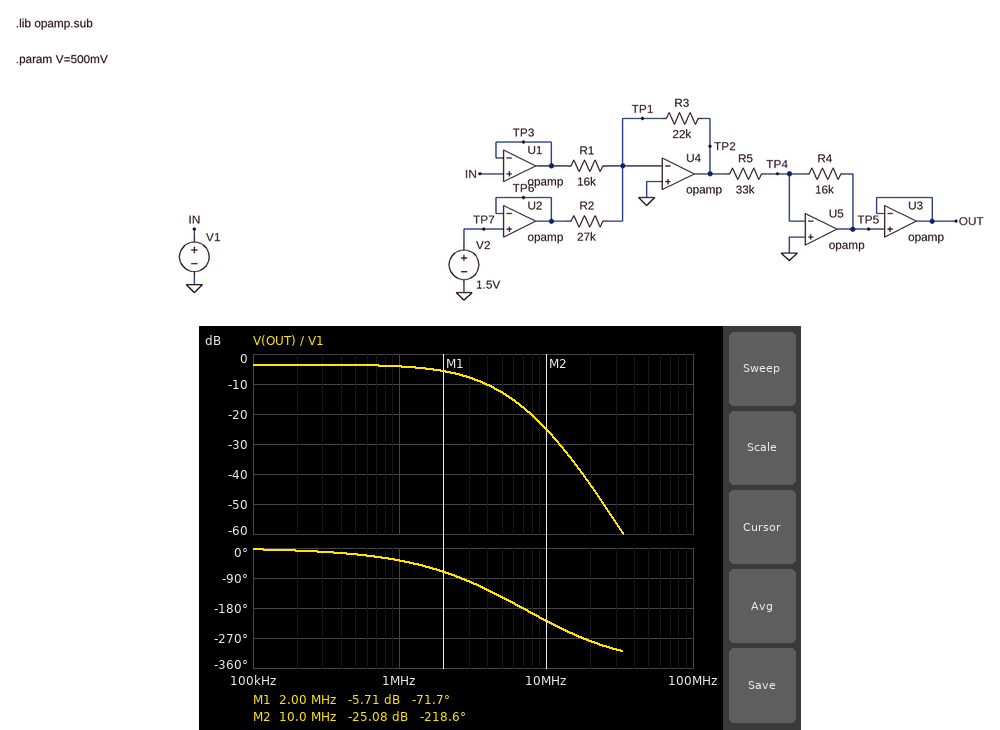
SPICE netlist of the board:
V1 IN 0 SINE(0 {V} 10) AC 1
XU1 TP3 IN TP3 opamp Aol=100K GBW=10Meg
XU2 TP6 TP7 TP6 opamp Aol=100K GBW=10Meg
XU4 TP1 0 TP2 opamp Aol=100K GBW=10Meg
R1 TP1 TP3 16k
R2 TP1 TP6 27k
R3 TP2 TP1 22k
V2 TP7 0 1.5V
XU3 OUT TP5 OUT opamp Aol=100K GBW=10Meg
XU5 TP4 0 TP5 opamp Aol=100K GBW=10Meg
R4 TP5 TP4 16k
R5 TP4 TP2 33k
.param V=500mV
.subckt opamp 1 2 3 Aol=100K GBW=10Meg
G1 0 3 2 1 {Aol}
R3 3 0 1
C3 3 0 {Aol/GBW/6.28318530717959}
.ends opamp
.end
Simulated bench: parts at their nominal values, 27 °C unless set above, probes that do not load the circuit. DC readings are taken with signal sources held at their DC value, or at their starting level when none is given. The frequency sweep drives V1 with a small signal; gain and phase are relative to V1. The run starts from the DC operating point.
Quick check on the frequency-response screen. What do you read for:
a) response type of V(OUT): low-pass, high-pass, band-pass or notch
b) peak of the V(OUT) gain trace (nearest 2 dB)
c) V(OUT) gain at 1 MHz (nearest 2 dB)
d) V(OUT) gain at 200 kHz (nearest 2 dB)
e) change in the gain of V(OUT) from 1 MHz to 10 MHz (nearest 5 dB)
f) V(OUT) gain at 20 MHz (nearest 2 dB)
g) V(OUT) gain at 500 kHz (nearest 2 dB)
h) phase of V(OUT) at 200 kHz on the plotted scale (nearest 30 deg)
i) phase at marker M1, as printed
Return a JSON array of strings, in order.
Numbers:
["low-pass", "-4 dB", "-4 dB", "-4 dB", "-20 dB", "-44 dB", "-4 dB", "0 deg", "-71.7 deg"]
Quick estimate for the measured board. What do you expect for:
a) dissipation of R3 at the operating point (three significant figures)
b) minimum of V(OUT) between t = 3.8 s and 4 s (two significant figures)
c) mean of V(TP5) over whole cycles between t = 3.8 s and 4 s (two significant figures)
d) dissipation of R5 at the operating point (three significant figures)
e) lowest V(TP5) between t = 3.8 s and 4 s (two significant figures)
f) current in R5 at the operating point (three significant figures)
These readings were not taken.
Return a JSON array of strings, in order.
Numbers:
["67.9 µW", "260 mV", "590 mV", "45.3 µW", "260 mV", "37.0 µA"]
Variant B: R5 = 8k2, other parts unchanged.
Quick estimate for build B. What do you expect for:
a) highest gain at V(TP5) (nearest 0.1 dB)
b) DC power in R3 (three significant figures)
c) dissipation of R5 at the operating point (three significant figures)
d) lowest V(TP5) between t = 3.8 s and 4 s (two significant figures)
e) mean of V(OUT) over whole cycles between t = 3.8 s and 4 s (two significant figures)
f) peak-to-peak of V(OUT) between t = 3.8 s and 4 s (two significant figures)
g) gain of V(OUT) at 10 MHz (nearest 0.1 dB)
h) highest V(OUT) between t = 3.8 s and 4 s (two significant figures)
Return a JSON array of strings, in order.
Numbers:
["8.6 dB", "67.9 µW", "182 µW", "1.0 V", "2.4 V", "2.7 V", "-17.8 dB", "3.7 V"]
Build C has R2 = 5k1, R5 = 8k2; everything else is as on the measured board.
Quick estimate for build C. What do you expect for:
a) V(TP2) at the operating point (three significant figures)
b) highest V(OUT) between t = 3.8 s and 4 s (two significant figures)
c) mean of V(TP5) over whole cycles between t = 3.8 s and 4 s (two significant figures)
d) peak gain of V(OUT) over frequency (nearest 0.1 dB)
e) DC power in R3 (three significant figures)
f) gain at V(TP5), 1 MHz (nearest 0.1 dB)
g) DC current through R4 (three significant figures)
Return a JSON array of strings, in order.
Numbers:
["-6.47 V", "14 V", "13 V", "8.6 dB", "1.90 mW", "6.6 dB", "789 µA"]
